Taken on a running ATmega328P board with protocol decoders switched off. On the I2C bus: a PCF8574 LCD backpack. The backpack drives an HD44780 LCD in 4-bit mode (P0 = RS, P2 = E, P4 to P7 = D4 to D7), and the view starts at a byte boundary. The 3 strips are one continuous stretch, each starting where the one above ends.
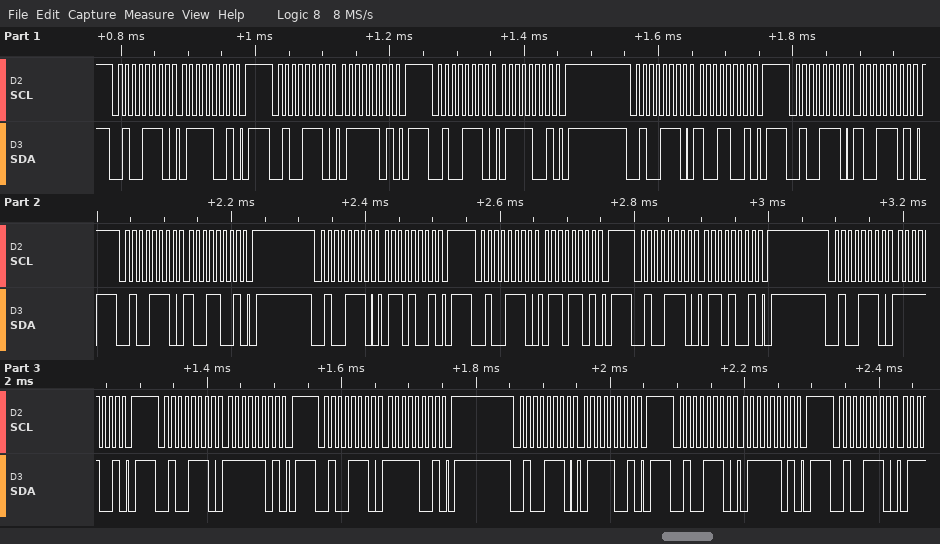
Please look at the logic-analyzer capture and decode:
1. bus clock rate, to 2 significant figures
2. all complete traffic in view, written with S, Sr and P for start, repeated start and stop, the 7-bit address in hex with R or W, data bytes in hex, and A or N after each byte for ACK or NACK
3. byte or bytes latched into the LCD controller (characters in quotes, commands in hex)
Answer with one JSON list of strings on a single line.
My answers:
["100 kHz", "S 27W A 79 A P S 27W A 7D A P S 27W A 79 A P S 27W A 99 A P S 27W A 9D A P S 27W A 99 A P S 27W A 69 A P S 27W A 6D A P S 27W A 69 A P S 27W A F9 A P S 27W A FD A P S 27W A F9 A P S 27W A 79 A P S 27W A 7D A P S 27W A", "'y' 'o'"]
